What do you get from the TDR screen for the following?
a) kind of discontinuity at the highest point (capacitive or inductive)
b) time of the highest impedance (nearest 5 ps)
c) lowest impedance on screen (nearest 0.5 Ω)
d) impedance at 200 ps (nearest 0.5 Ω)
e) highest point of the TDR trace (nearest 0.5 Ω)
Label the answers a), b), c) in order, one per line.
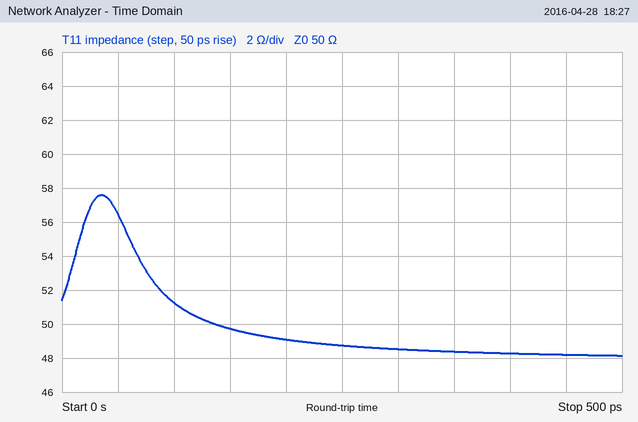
a) inductive
b) 35 ps
c) 48.0 Ω
d) 49.0 Ω
e) 57.5 Ω
